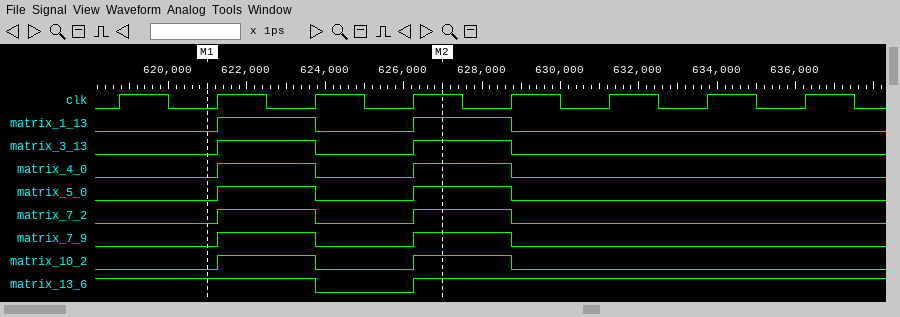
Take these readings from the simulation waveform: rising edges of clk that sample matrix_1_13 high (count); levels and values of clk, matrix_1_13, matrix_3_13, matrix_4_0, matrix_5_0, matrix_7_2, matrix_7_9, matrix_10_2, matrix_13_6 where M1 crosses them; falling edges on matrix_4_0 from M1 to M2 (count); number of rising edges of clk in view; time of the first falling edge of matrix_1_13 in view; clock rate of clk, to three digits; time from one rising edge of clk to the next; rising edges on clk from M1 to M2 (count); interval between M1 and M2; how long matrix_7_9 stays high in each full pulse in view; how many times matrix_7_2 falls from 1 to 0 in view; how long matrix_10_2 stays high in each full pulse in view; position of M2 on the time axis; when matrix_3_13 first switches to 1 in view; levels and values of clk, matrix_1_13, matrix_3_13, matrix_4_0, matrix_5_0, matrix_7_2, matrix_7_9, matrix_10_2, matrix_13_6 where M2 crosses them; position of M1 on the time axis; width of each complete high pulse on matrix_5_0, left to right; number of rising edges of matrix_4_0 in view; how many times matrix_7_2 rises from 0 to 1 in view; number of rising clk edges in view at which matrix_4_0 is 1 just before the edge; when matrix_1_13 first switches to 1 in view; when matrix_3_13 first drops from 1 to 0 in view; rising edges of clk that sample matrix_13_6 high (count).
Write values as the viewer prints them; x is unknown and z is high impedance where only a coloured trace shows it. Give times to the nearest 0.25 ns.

2
clk=0, matrix_1_13=0, matrix_3_13=0, matrix_4_0=0, matrix_5_0=0, matrix_7_2=0, matrix_7_9=0, matrix_10_2=0, matrix_13_6=1
1
8
623.75 ns
400 MHz
2.5 ns
3
6 ns
2.5 ns, 2.5 ns
2
2.5 ns, 2.5 ns
627 ns
621.25 ns
clk=1, matrix_1_13=1, matrix_3_13=1, matrix_4_0=1, matrix_5_0=1, matrix_7_2=1, matrix_7_9=1, matrix_10_2=1, matrix_13_6=1
621 ns
2.5 ns, 2.5 ns
2
2
2
621.25 ns
623.75 ns
7
